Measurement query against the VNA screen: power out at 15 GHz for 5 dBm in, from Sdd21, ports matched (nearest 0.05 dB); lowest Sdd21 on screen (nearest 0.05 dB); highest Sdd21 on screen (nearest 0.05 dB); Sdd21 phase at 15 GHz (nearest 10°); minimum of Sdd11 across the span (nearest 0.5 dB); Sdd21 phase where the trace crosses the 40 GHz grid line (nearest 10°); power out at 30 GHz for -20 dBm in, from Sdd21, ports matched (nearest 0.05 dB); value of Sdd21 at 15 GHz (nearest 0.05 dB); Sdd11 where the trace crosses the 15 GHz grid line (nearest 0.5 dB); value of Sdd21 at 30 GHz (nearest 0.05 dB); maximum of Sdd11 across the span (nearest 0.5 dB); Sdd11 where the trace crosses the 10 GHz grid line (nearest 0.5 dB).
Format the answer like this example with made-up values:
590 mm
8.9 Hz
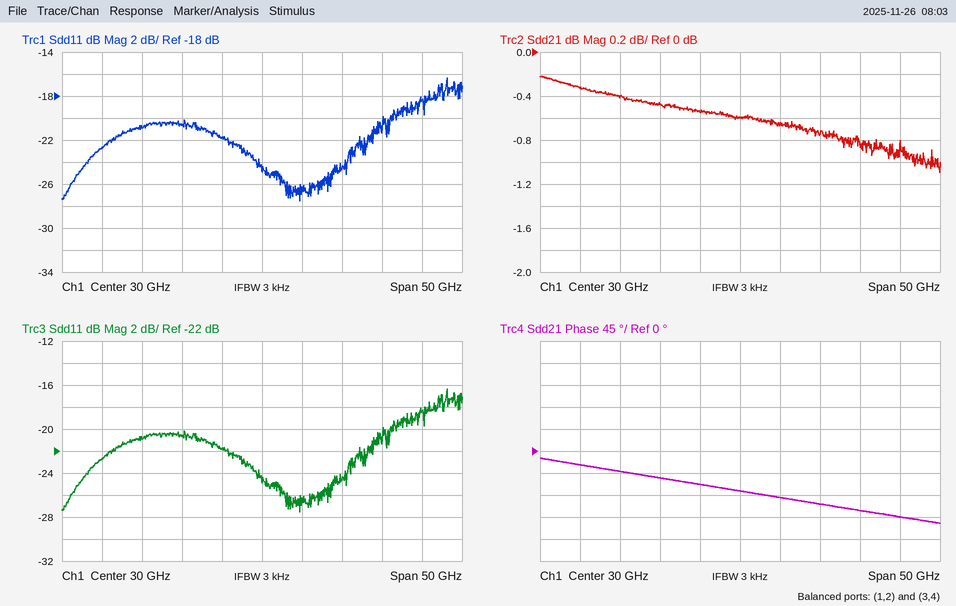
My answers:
4.60 dBm
-1.10 dB
-0.20 dB
-40°
-27.5 dB
-110°
-20.60 dBm
-0.40 dB
-21.0 dB
-0.60 dB
-16.5 dB
-22.5 dB
